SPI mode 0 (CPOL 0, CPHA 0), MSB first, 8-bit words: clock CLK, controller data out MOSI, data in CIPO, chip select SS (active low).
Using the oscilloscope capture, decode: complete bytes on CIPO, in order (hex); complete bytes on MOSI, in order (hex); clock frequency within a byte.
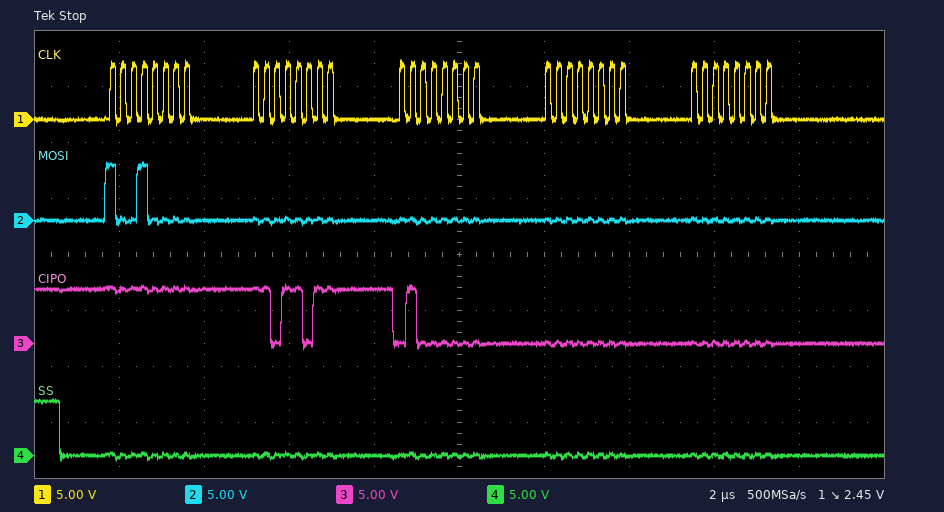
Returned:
FF DB 40 00 00
90 00 00 00 00
4 MHz
